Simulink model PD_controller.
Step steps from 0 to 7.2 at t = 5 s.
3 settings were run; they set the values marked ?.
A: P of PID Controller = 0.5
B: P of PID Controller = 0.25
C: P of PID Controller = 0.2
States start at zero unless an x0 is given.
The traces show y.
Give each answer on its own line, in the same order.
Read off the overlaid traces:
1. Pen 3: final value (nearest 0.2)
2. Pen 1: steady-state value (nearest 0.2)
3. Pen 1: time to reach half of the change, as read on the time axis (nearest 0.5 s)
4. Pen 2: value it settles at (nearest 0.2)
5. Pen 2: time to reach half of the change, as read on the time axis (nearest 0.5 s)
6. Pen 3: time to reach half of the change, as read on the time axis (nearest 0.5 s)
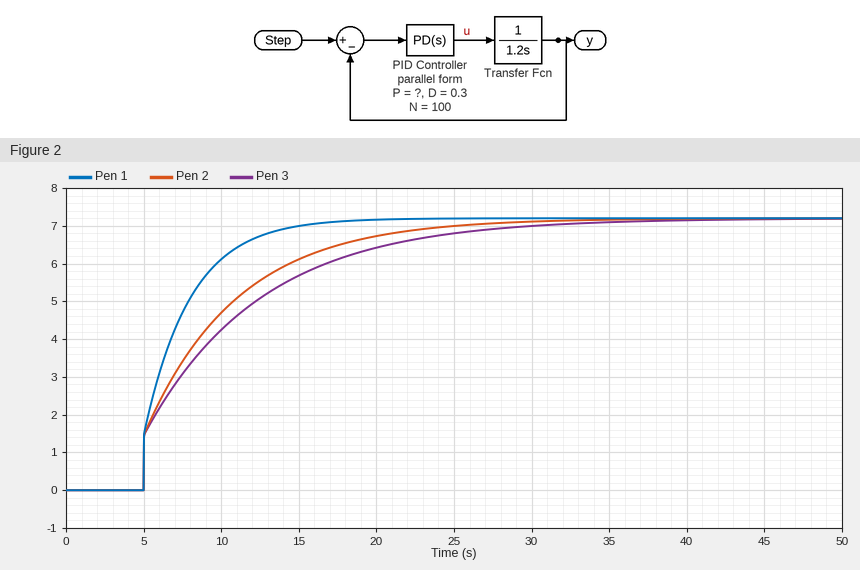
7.2
7.2
6.5 s
7.2
8.0 s
8.5 s
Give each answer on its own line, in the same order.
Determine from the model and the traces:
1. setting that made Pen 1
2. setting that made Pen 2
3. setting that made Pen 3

A
B
C
